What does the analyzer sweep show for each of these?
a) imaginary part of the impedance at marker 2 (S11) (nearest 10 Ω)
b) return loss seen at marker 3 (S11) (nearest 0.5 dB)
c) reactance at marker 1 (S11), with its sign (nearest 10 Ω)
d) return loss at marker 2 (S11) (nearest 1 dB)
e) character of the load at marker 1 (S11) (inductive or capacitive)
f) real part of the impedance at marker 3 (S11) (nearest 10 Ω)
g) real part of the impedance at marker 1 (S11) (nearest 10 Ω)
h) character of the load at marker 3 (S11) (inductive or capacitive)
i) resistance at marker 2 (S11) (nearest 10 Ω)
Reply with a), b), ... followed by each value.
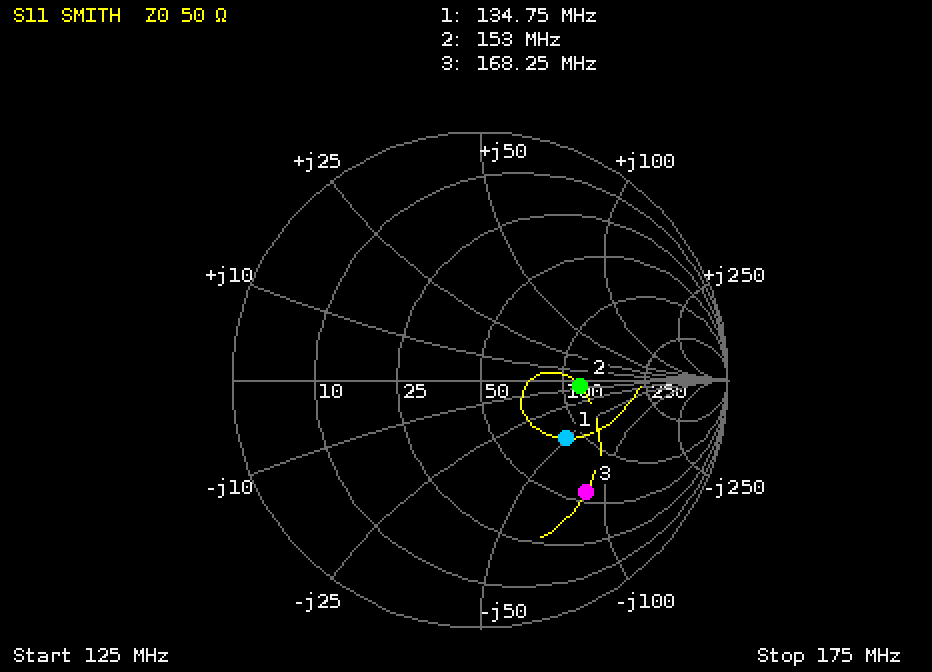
a) -10 Ω
b) 4.0 dB
c) -50 Ω
d) 8 dB
e) capacitive
f) 60 Ω
g) 90 Ω
h) capacitive
i) 120 Ω
